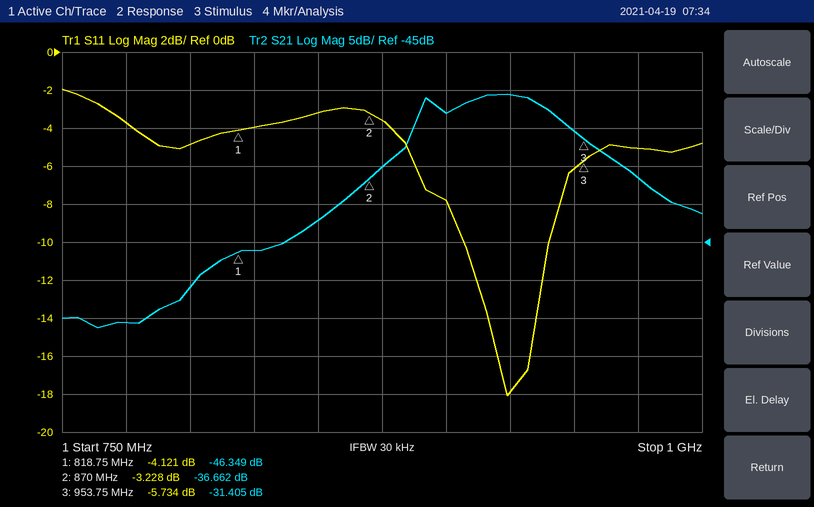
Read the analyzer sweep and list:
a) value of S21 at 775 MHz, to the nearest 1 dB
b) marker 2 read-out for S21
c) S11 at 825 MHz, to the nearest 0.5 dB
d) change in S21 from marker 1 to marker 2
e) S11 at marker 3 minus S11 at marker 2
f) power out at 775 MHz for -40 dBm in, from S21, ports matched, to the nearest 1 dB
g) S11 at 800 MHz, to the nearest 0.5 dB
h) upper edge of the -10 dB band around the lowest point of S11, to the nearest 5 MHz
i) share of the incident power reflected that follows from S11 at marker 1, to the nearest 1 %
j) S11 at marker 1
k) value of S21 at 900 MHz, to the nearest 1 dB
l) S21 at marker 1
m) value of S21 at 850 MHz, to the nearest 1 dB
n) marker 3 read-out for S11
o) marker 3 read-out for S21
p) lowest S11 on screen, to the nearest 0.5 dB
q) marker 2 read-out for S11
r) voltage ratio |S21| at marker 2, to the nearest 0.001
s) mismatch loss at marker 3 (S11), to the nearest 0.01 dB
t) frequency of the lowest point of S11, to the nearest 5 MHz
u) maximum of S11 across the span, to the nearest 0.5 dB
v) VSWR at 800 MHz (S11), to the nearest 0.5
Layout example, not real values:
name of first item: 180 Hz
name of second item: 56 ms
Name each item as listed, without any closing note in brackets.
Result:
value of S21 at 775 MHz, to the nearest 1 dB: -56 dB
marker 2 read-out for S21: -36.662 dB
S11 at 825 MHz, to the nearest 0.5 dB: -4.0 dB
change in S21 from marker 1 to marker 2: 9.687 dB
S11 at marker 3 minus S11 at marker 2: -2.506 dB
power out at 775 MHz for -40 dBm in, from S21, ports matched, to the nearest 1 dB: -96 dBm
S11 at 800 MHz, to the nearest 0.5 dB: -5.0 dB
upper edge of the -10 dB band around the lowest point of S11, to the nearest 5 MHz: 940 MHz
share of the incident power reflected that follows from S11 at marker 1, to the nearest 1 %: 39 %
S11 at marker 1: -4.121 dB
value of S21 at 900 MHz, to the nearest 1 dB: -28 dB
S21 at marker 1: -46.349 dB
value of S21 at 850 MHz, to the nearest 1 dB: -42 dB
marker 3 read-out for S11: -5.734 dB
marker 3 read-out for S21: -31.405 dB
lowest S11 on screen, to the nearest 0.5 dB: -18.0 dB
marker 2 read-out for S11: -3.228 dB
voltage ratio |S21| at marker 2, to the nearest 0.001: 0.015
mismatch loss at marker 3 (S11), to the nearest 0.01 dB: 1.35 dB
frequency of the lowest point of S11, to the nearest 5 MHz: 925 MHz
maximum of S11 across the span, to the nearest 0.5 dB: -2.0 dB
VSWR at 800 MHz (S11), to the nearest 0.5: 3.5
